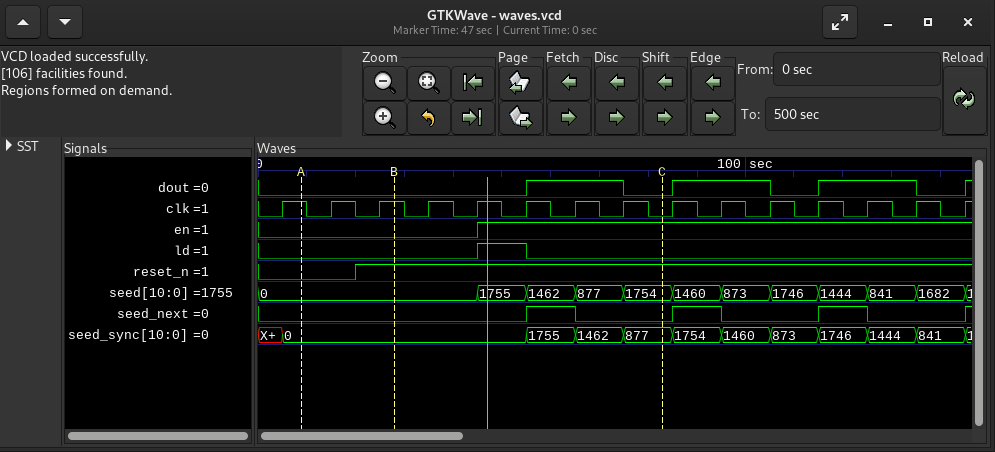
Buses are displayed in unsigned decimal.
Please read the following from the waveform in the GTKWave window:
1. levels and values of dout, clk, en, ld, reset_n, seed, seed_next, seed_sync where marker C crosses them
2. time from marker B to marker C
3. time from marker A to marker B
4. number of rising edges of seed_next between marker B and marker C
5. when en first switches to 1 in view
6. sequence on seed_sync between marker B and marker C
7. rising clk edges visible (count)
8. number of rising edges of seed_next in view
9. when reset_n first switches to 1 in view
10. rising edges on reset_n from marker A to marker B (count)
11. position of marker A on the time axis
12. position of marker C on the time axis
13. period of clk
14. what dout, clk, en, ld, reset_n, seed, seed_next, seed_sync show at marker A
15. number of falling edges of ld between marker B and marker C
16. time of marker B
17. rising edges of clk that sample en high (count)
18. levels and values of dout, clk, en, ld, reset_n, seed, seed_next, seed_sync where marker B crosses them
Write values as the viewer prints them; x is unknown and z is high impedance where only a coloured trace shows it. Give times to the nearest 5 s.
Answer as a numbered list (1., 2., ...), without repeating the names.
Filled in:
1. dout=0, clk=0, en=1, ld=0, reset_n=1, seed=1754, seed_next=0, seed_sync=877
2. 55 s
3. 20 s
4. 1
5. 45 s
6. 0, 1755, 1462, 877
7. 15
8. 4
9. 20 s
10. 1
11. 10 s
12. 85 s
13. 10 s
14. dout=0, clk=1, en=0, ld=0, reset_n=0, seed=0, seed_next=0, seed_sync=0
15. 1
16. 30 s
17. 10
18. dout=0, clk=1, en=0, ld=0, reset_n=1, seed=0, seed_next=0, seed_sync=0
